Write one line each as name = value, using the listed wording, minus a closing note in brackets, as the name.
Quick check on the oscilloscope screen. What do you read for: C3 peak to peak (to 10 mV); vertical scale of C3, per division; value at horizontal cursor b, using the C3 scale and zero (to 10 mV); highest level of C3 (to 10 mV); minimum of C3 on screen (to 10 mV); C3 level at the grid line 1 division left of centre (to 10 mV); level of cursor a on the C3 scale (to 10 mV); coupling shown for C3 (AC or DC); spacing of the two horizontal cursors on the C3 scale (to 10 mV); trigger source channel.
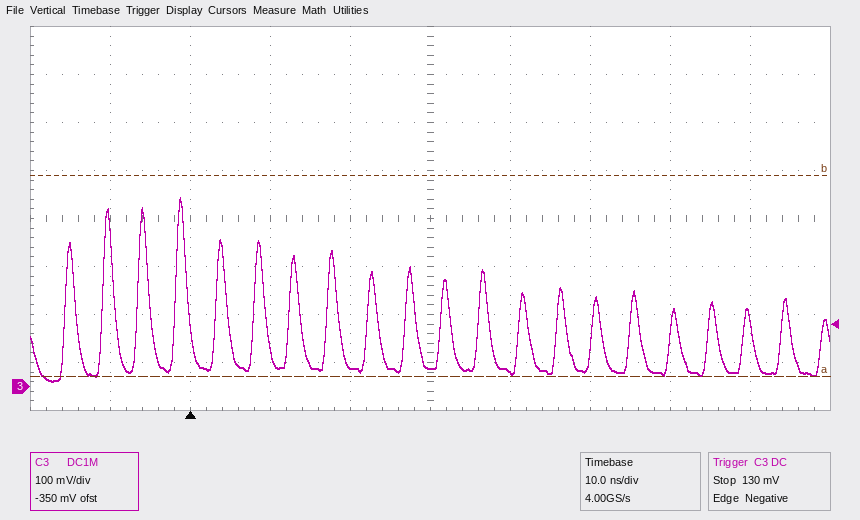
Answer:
C3 peak to peak = 380 mV
vertical scale of C3, per division = 100 mV
value at horizontal cursor b, using the C3 scale and zero = 440 mV
highest level of C3 = 390 mV
minimum of C3 on screen = 10 mV
C3 level at the grid line 1 division left of centre = 40 mV
level of cursor a on the C3 scale = 20 mV
coupling shown for C3 = DC
spacing of the two horizontal cursors on the C3 scale = 420 mV
trigger source channel = C3
